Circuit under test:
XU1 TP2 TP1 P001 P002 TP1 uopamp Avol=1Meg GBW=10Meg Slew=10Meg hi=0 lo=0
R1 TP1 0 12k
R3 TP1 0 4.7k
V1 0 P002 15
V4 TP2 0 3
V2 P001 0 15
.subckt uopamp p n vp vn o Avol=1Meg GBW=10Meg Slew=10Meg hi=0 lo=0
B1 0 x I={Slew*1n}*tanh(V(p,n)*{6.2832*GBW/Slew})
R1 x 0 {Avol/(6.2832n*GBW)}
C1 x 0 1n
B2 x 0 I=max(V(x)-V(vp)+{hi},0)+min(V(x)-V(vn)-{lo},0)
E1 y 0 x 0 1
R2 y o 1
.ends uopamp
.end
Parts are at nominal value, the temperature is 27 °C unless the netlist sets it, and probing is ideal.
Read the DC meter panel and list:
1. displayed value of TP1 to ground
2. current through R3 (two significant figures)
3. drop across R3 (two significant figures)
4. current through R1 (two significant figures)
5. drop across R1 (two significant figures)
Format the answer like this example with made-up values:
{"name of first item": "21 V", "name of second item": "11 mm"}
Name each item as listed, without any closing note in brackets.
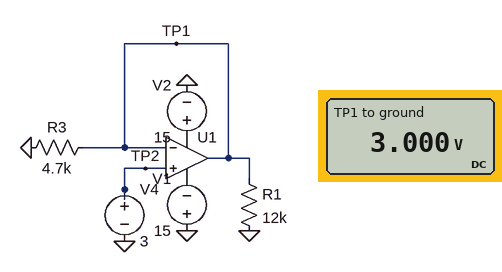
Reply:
{"displayed value of TP1 to ground": "3.000 V", "current through R3": "640 µA", "drop across R3": "3.0 V", "current through R1": "250 µA", "drop across R1": "3.0 V"}
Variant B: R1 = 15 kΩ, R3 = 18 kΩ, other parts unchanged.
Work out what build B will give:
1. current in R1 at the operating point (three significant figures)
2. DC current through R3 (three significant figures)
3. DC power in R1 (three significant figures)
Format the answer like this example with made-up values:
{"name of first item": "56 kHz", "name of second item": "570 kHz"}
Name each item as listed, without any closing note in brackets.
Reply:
{"current in R1 at the operating point": "200 µA", "DC current through R3": "167 µA", "DC power in R1": "600 µW"}
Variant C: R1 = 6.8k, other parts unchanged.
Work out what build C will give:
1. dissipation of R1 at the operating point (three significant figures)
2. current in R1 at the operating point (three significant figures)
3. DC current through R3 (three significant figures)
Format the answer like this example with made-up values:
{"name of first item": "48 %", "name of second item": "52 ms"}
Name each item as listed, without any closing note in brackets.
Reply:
{"dissipation of R1 at the operating point": "1.32 mW", "current in R1 at the operating point": "441 µA", "DC current through R3": "638 µA"}
